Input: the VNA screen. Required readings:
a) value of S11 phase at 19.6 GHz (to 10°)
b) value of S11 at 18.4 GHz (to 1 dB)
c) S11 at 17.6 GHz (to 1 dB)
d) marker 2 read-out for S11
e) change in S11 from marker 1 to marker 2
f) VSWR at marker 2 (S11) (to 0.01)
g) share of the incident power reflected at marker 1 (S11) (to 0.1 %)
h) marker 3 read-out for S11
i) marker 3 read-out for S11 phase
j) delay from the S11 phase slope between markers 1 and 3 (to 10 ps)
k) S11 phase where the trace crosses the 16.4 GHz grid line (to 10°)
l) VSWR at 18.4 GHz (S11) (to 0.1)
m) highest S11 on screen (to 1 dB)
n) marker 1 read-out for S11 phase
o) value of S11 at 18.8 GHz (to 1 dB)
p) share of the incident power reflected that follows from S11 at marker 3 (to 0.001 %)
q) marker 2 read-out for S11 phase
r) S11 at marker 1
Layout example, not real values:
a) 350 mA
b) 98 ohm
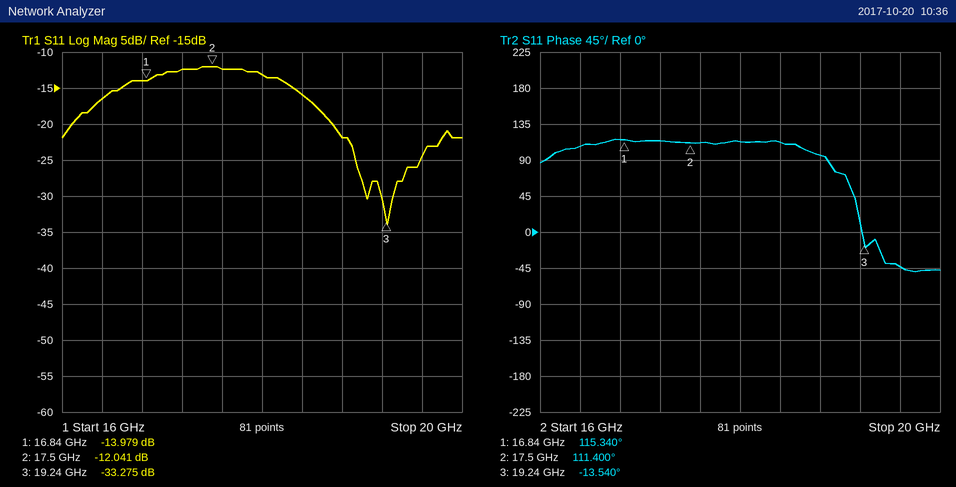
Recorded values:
a) -40°
b) -16 dB
c) -12 dB
d) -12.041 dB
e) 1.938 dB
f) 1.67
g) 4.0 %
h) -33.275 dB
i) -13.540°
j) 150 ps
k) 110°
l) 1.4
m) -12 dB
n) 115.340°
o) -22 dB
p) 0.047 %
q) 111.400°
r) -13.979 dB
